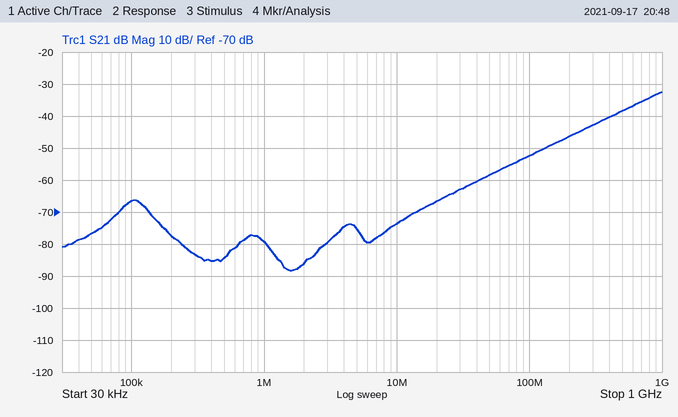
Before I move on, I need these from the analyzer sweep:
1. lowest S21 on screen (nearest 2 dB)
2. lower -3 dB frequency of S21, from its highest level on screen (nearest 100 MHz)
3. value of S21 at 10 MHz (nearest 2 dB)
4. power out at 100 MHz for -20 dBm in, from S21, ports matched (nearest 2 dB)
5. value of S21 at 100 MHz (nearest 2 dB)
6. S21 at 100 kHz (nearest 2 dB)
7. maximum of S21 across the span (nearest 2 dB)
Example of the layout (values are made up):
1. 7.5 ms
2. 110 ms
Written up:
1. -88 dB
2. 700 MHz
3. -74 dB
4. -72 dBm
5. -52 dB
6. -66 dB
7. -32 dB
